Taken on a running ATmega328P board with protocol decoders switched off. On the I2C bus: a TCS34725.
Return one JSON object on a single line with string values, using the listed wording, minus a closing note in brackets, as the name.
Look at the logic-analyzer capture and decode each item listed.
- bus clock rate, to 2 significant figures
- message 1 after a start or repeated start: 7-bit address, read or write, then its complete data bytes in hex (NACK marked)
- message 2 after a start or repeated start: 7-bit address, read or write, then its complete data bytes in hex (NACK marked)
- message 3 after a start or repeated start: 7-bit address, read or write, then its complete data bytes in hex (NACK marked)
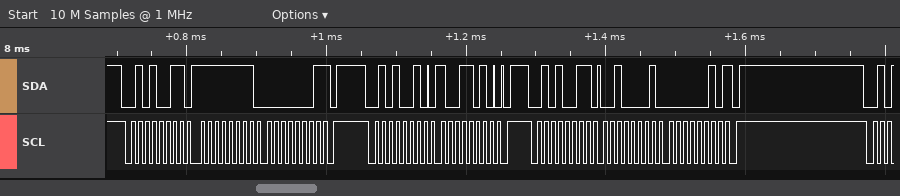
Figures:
{"bus clock rate, to 2 significant figures": "100 kHz", "message 1 after a start or repeated start: 7-bit address, read or write, then its complete data bytes in hex": "0x29 read: FF 01 NACK", "message 2 after a start or repeated start: 7-bit address, read or write, then its complete data bytes in hex": "0x29 write: 9A", "message 3 after a start or repeated start: 7-bit address, read or write, then its complete data bytes in hex": "0x29 read: 21 02 NACK"}
